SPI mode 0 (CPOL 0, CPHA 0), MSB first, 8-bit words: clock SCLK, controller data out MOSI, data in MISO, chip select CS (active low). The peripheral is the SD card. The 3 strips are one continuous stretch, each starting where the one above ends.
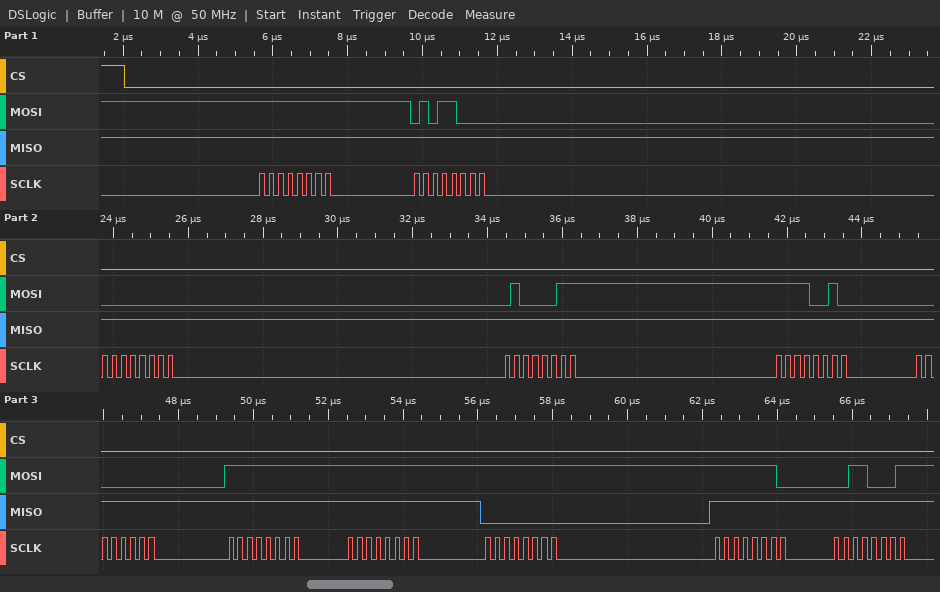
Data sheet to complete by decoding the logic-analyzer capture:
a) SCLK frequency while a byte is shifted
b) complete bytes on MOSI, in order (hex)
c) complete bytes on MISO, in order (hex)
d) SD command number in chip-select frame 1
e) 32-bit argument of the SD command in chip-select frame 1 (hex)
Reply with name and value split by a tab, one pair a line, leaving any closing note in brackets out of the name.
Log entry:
SCLK frequency while a byte is shifted	4 MHz
complete bytes on MOSI, in order	0xFF 0x58 0x00 0x43 0xF2 0x00 0xFF 0xFF 0xFF 0xFE 0x31
complete bytes on MISO, in order	0xFF 0xFF 0xFF 0xFF 0xFF 0xFF 0xFF 0xFF 0x00 0xFF 0xFF
SD command number in chip-select frame 1	CMD24
32-bit argument of the SD command in chip-select frame 1	0x0043F200
